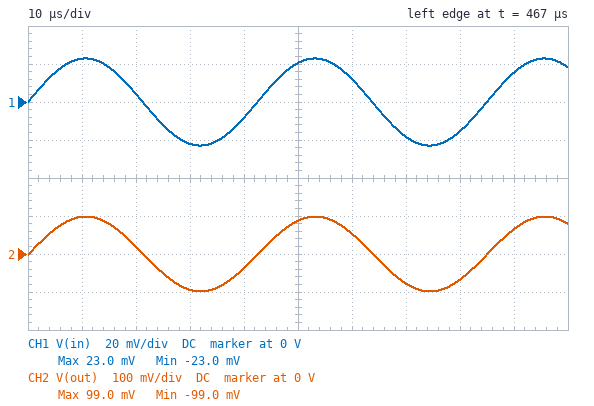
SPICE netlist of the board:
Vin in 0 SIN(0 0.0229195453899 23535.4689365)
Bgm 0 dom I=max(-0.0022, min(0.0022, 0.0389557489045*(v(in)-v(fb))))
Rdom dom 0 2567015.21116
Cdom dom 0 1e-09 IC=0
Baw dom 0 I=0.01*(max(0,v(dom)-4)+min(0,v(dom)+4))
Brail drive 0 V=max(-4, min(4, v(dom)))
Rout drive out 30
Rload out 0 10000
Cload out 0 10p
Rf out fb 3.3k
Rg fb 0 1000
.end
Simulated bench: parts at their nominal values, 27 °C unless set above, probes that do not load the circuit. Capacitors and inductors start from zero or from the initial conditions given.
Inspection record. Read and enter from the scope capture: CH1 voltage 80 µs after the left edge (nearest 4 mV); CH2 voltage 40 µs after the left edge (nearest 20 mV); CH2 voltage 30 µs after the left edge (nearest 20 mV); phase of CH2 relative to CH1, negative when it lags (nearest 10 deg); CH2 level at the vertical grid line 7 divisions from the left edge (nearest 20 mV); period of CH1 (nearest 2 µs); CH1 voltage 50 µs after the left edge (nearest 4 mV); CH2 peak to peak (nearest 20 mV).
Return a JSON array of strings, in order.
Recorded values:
["-16 mV", "-40 mV", "-100 mV", "0 deg", "-80 mV", "42 µs", "20 mV", "200 mV"]
